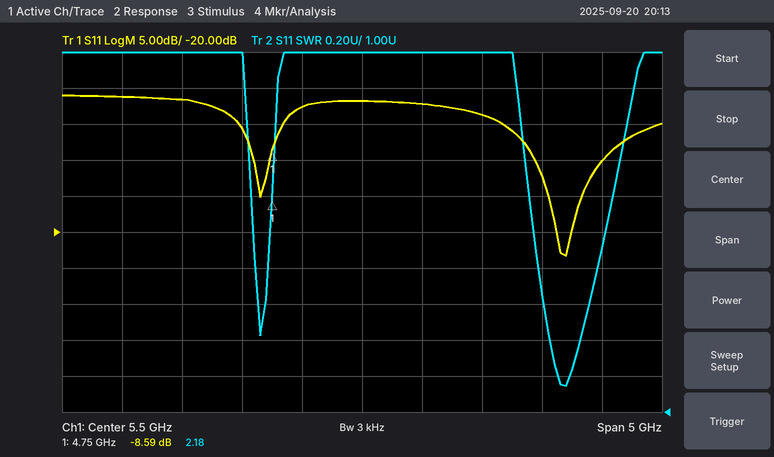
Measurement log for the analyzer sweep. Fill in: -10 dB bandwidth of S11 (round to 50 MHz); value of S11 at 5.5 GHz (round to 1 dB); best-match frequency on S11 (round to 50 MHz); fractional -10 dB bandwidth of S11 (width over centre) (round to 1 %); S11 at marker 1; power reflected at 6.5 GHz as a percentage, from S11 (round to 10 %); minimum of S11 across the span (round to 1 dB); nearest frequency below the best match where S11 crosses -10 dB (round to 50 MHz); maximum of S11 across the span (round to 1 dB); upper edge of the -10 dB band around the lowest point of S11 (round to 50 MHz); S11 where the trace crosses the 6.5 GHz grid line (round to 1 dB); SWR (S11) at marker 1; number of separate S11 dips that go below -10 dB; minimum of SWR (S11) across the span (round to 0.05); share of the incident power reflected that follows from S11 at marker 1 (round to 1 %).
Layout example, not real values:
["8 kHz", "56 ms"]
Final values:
["550 MHz", "-2 dB", "7.20 GHz", "8 %", "-8.59 dB", "40 %", "-23 dB", "6.95 GHz", "-1 dB", "7.50 GHz", "-4 dB", "2.18", "2", "1.15", "14 %"]
